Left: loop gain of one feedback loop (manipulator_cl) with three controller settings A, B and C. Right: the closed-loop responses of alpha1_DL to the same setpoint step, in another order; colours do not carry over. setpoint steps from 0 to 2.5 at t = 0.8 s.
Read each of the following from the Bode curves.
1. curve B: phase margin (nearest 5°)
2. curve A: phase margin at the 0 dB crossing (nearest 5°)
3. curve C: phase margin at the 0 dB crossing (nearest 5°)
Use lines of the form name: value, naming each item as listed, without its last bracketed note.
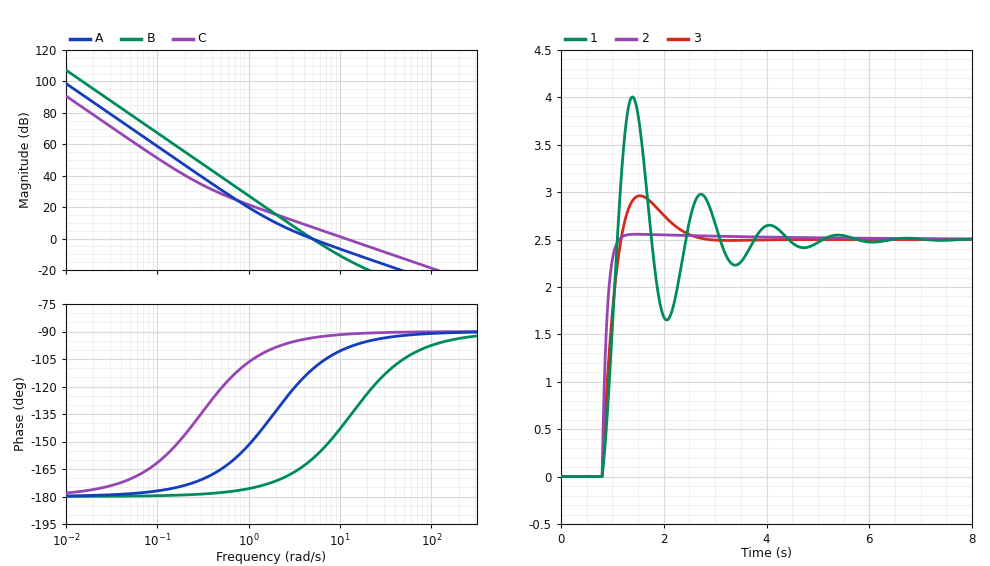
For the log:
curve B: phase margin: 20°
curve A: phase margin at the 0 dB crossing: 70°
curve C: phase margin at the 0 dB crossing: 90°
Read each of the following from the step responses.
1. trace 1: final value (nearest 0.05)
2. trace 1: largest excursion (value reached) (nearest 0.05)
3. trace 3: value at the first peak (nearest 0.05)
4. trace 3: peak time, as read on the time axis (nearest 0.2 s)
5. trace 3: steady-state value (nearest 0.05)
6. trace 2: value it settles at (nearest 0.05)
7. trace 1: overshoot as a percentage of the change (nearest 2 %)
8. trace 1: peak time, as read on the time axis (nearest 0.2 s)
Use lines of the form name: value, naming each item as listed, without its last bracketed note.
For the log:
trace 1: final value: 2.50
trace 1: largest excursion (value reached): 4.00
trace 3: value at the first peak: 2.95
trace 3: peak time, as read on the time axis: 1.6 s
trace 3: steady-state value: 2.50
trace 2: value it settles at: 2.50
trace 1: overshoot as a percentage of the change: 60 %
trace 1: peak time, as read on the time axis: 1.4 s
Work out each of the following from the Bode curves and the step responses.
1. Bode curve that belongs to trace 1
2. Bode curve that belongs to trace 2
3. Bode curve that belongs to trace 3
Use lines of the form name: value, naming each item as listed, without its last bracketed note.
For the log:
Bode curve that belongs to trace 1: B
Bode curve that belongs to trace 2: C
Bode curve that belongs to trace 3: A
